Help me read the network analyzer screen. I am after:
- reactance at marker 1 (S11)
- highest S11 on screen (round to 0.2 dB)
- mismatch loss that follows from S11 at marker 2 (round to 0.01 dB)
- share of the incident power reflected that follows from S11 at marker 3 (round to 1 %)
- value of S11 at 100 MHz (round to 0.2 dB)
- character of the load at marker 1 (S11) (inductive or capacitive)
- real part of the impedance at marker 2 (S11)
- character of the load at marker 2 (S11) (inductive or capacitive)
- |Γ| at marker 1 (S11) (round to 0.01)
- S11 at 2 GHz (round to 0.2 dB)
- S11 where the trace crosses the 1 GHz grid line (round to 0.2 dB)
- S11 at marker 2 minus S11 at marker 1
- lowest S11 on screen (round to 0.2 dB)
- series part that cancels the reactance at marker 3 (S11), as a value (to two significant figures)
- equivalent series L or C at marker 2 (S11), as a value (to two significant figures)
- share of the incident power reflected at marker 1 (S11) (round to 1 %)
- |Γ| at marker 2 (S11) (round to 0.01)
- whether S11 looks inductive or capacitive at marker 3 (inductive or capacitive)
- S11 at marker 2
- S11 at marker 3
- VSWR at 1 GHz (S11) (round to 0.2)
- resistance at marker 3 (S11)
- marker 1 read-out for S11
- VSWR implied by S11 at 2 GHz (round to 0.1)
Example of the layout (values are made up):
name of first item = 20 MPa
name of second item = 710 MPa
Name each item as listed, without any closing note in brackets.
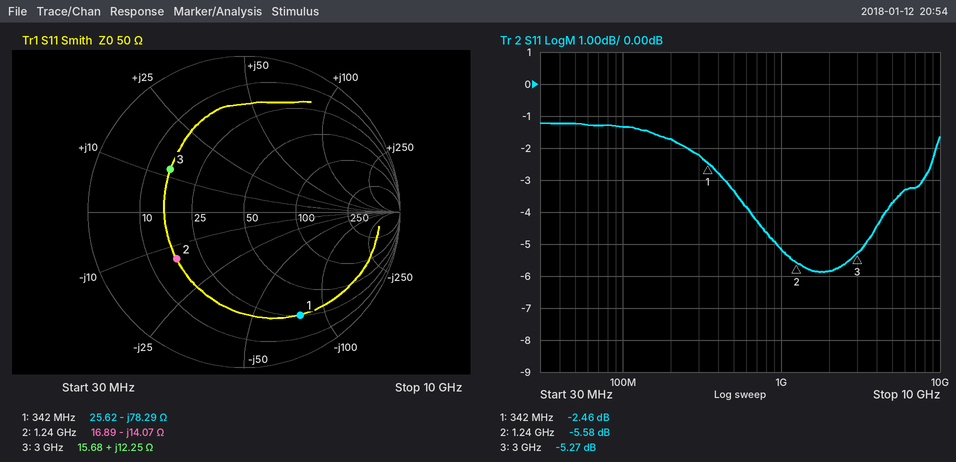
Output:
reactance at marker 1 = -78.29 Ω
highest S11 on screen = -1.2 dB
mismatch loss that follows from S11 at marker 2 = 1.41 dB
share of the incident power reflected that follows from S11 at marker 3 = 30 %
value of S11 at 100 MHz = -1.4 dB
character of the load at marker 1 (S11) = capacitive
real part of the impedance at marker 2 = 16.89 Ω
character of the load at marker 2 (S11) = capacitive
|Γ| at marker 1 (S11) = 0.75
S11 at 2 GHz = -5.8 dB
S11 where the trace crosses the 1 GHz grid line = -5.2 dB
S11 at marker 2 minus S11 at marker 1 = -3.12 dB
lowest S11 on screen = -5.8 dB
series part that cancels the reactance at marker 3 (S11), as a value = 4.3 pF
equivalent series L or C at marker 2 (S11), as a value = 9.1 pF
share of the incident power reflected at marker 1 (S11) = 57 %
|Γ| at marker 2 (S11) = 0.53
whether S11 looks inductive or capacitive at marker 3 = inductive
S11 at marker 2 = -5.58 dB
S11 at marker 3 = -5.27 dB
VSWR at 1 GHz (S11) = 3.4
resistance at marker 3 = 15.68 Ω
marker 1 read-out for S11 = -2.46 dB
VSWR implied by S11 at 2 GHz = 3.1
